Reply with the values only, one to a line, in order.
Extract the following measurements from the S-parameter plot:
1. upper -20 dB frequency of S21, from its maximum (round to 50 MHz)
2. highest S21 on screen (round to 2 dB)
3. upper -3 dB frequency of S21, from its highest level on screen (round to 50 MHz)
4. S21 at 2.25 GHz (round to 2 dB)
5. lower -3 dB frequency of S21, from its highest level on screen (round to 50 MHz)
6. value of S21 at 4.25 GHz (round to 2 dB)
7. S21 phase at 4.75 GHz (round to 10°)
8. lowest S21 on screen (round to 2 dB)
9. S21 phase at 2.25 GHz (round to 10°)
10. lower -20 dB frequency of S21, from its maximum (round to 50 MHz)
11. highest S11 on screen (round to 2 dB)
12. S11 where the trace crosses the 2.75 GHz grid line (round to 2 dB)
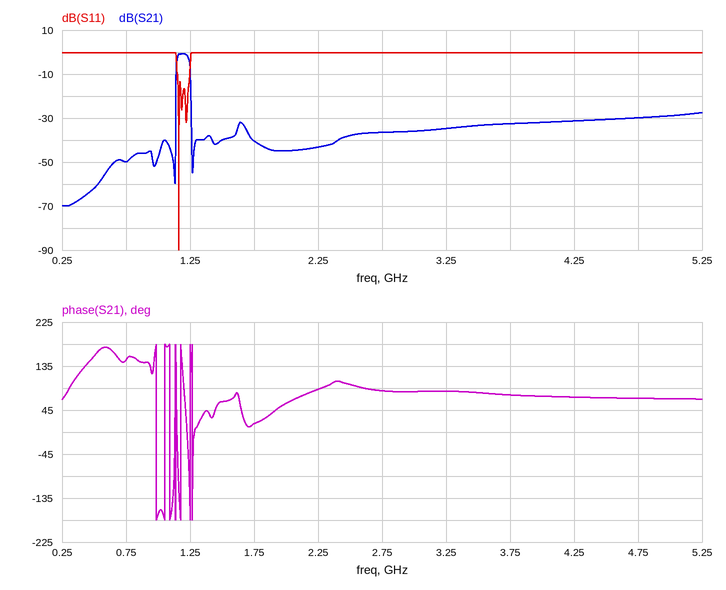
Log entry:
1.25 GHz
0 dB
1.25 GHz
-44 dB
1.15 GHz
-32 dB
70°
-70 dB
90°
1.15 GHz
0 dB
0 dB
